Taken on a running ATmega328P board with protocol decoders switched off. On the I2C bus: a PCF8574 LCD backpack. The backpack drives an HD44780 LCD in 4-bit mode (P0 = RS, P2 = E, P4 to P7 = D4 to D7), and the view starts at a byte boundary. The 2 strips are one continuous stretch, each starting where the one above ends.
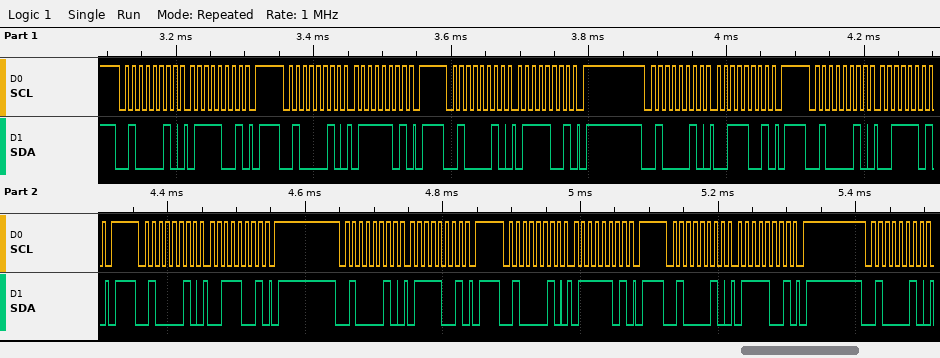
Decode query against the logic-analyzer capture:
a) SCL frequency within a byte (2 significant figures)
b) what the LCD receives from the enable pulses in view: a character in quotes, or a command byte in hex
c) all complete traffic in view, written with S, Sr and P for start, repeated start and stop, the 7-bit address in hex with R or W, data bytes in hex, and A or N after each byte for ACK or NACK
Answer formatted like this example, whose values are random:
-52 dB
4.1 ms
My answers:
100 kHz
's'
S 21W A 79 A P S 21W A 7D A P S 21W A 79 A P S 21W A 39 A P S 21W A 3D A P S 21W A 39 A P S 21W A 79 A P S 21W A 7D A P S 21W A 79 A P S 21W A
